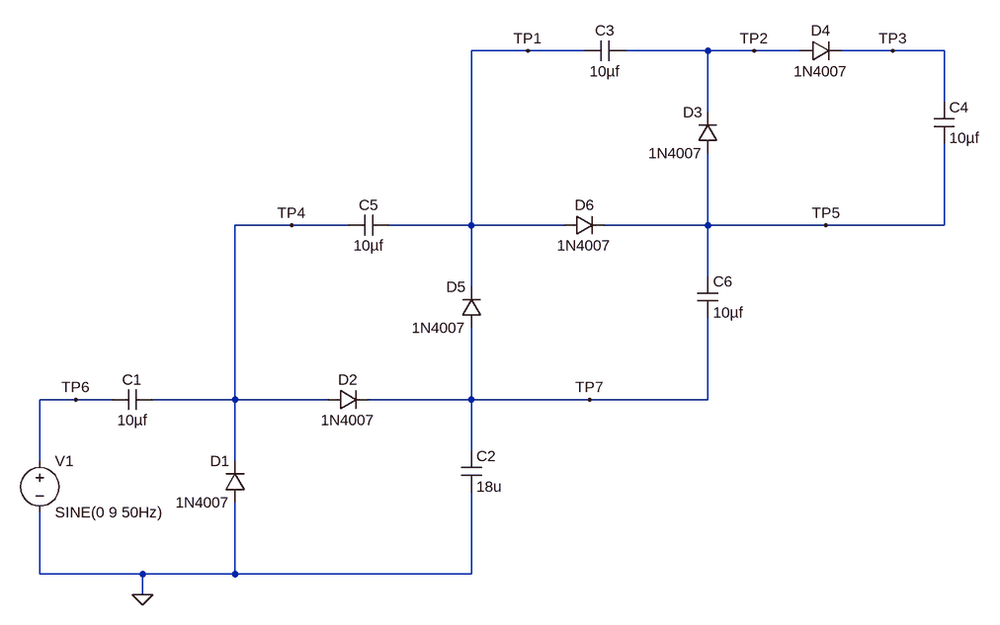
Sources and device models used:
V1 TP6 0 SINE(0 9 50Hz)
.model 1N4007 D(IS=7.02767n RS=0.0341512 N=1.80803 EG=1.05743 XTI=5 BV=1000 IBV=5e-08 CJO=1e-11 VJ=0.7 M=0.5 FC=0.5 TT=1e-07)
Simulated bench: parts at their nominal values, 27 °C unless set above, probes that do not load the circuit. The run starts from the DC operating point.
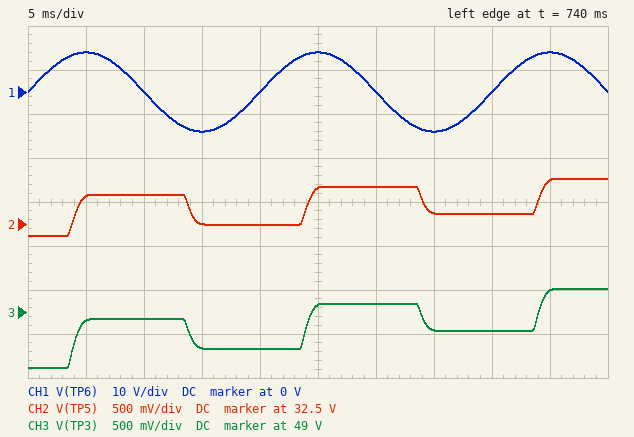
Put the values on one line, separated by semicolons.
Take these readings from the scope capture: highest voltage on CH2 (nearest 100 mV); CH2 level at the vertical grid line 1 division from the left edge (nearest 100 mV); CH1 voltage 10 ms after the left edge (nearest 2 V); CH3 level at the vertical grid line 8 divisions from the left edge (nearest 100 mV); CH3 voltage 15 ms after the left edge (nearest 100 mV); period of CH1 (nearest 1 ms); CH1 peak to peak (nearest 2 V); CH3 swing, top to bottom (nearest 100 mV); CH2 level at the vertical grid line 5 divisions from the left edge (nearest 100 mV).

33.0 V; 32.8 V; 0 V; 48.8 V; 48.6 V; 20 ms; 18 V; 900 mV; 32.9 V
